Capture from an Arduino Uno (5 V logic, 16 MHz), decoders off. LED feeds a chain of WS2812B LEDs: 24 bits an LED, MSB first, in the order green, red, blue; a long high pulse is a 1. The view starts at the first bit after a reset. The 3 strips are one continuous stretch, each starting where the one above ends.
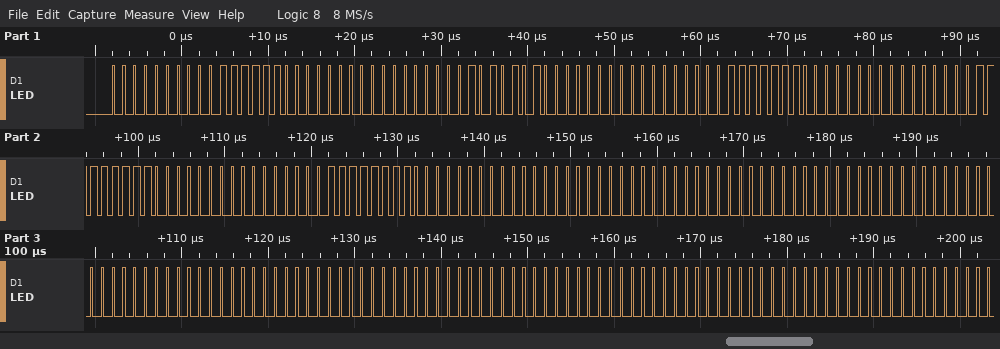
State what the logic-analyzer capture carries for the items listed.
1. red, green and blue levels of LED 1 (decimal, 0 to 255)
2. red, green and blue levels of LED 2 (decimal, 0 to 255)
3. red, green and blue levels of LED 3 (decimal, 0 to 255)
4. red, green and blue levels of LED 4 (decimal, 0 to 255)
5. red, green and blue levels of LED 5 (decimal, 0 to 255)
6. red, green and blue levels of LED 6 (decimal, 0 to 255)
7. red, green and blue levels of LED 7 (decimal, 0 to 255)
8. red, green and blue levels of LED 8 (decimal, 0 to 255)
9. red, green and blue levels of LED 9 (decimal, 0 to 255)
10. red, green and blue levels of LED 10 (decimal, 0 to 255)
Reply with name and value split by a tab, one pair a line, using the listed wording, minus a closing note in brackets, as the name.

red, green and blue levels of LED 1	63, 0, 0
red, green and blue levels of LED 2	85, 0, 0
red, green and blue levels of LED 3	127, 0, 0
red, green and blue levels of LED 4	255, 0, 0
red, green and blue levels of LED 5	255, 0, 0
red, green and blue levels of LED 6	0, 0, 0
red, green and blue levels of LED 7	0, 0, 0
red, green and blue levels of LED 8	0, 0, 0
red, green and blue levels of LED 9	0, 0, 0
red, green and blue levels of LED 10	0, 0, 0
